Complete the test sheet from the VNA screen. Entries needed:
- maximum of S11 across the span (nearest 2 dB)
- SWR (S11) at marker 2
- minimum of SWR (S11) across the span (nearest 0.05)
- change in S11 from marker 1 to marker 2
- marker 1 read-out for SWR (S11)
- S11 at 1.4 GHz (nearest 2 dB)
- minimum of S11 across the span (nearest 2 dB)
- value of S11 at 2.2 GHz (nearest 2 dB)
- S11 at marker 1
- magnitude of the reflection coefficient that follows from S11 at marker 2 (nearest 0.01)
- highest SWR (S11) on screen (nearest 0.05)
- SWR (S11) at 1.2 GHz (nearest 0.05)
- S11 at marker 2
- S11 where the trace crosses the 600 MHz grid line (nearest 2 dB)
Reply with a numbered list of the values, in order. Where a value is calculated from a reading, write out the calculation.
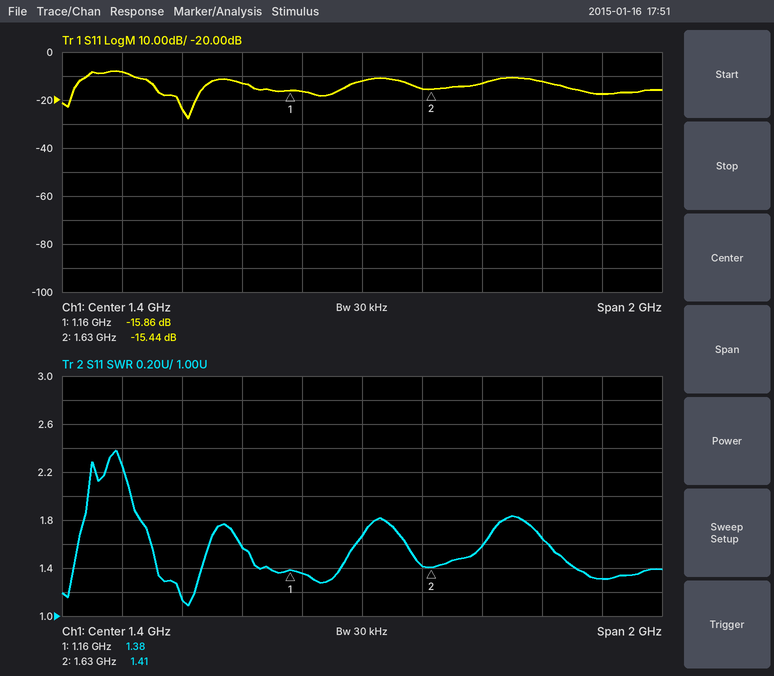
1. -8 dB
2. 1.41
3. 1.10
4. -15.44 − (-15.86) = 0.42 dB
5. 1.38
6. -12 dB
7. -28 dB
8. -18 dB
9. -15.86 dB
10. 10^(-15.44/20) ≈ 0.17
11. 2.40
12. 1.35
13. -15.44 dB
14. -8 dB
